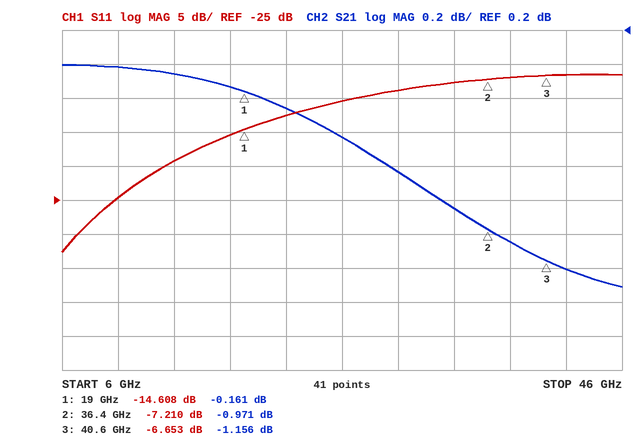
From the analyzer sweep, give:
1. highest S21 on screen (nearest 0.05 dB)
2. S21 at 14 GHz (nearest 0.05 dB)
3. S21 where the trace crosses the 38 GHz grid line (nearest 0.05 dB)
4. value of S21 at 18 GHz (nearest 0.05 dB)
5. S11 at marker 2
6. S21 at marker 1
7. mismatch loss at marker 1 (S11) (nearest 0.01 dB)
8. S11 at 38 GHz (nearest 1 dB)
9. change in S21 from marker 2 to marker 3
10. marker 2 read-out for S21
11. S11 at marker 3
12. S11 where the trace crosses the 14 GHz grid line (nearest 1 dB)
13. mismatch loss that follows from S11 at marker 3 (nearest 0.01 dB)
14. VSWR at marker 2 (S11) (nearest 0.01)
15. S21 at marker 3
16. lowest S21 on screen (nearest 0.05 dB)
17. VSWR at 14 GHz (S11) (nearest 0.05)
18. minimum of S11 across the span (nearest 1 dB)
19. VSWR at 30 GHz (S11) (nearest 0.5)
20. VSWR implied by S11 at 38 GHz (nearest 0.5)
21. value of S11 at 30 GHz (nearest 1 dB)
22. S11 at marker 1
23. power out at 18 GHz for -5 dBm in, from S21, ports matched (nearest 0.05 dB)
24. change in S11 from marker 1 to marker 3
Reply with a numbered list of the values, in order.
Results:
1. 0.00 dB
2. -0.05 dB
3. -1.05 dB
4. -0.15 dB
5. -7.210 dB
6. -0.161 dB
7. 0.15 dB
8. -7 dB
9. -0.185 dB
10. -0.971 dB
11. -6.653 dB
12. -19 dB
13. 1.06 dB
14. 2.55
15. -1.156 dB
16. -1.30 dB
17. 1.25
18. -33 dB
19. 2.0
20. 2.5
21. -9 dB
22. -14.608 dB
23. -5.15 dBm
24. 7.955 dB
